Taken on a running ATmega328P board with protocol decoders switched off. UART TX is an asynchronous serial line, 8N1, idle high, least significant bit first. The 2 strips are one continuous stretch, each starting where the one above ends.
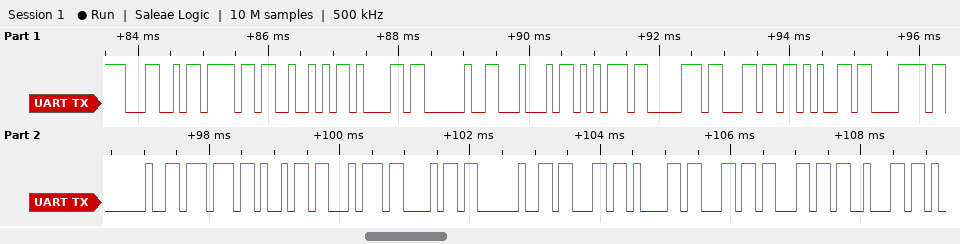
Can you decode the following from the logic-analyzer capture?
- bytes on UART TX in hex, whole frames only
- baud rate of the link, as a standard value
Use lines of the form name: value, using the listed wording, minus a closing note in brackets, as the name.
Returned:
bytes on UART TX in hex, whole frames only: 0x4C 0x6F 0x52 0x61 0x20 0x44 0x75 0x70 0x6C 0x65 0x78 0x20 0x77 0x69 0x74 0x68 0x20 0x63 0x61 0x6C 0x6C 0x62
baud rate of the link, as a standard value: 9600 baud
